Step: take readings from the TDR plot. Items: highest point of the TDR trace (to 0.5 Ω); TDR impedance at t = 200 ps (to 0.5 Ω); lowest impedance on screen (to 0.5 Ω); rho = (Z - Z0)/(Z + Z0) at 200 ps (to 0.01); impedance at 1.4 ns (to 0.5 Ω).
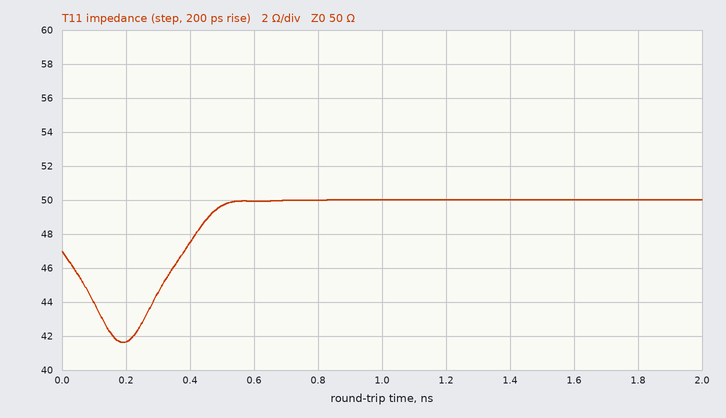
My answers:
50.0 Ω
41.5 Ω
41.5 Ω
-0.09
50.0 Ω
